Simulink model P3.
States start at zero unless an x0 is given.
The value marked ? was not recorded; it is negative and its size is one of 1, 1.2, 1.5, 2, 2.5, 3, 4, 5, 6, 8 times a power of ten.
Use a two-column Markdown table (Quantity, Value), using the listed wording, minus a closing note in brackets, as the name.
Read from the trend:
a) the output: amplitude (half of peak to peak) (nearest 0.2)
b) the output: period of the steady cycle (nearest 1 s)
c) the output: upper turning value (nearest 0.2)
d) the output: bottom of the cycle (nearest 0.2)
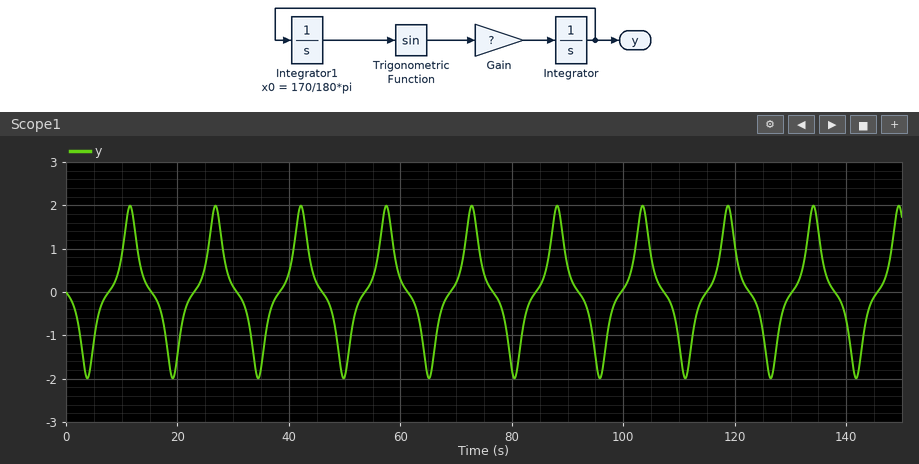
| Quantity | Value |
|---|---|
| the output: amplitude (half of peak to peak) | 2.0 |
| the output: period of the steady cycle | 15 s |
| the output: upper turning value | 2.0 |
| the output: bottom of the cycle | -2.0 |
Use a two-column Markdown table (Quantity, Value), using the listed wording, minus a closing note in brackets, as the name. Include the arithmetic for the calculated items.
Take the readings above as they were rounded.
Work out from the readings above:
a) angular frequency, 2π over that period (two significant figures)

| Quantity | Value |
|---|---|
| angular frequency, 2π over that period | 2π / 15 = 0.42 rad/s |
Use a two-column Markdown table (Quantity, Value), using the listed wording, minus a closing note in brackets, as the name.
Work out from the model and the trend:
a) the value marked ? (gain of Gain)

| Quantity | Value |
|---|---|
| the value marked ? | -1 |
